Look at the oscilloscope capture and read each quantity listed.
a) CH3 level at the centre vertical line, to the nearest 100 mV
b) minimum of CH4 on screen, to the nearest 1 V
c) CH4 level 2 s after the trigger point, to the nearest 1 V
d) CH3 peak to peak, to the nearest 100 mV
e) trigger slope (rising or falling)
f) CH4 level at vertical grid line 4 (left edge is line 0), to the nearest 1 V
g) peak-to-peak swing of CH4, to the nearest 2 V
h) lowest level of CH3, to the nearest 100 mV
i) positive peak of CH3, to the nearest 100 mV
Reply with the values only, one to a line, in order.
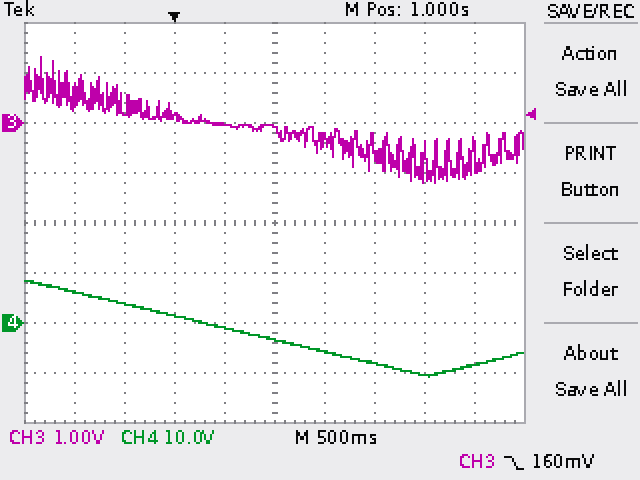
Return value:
-100 mV
-11 V
-8 V
2.5 V
falling
-1 V
20 V
-1.2 V
1.3 V
